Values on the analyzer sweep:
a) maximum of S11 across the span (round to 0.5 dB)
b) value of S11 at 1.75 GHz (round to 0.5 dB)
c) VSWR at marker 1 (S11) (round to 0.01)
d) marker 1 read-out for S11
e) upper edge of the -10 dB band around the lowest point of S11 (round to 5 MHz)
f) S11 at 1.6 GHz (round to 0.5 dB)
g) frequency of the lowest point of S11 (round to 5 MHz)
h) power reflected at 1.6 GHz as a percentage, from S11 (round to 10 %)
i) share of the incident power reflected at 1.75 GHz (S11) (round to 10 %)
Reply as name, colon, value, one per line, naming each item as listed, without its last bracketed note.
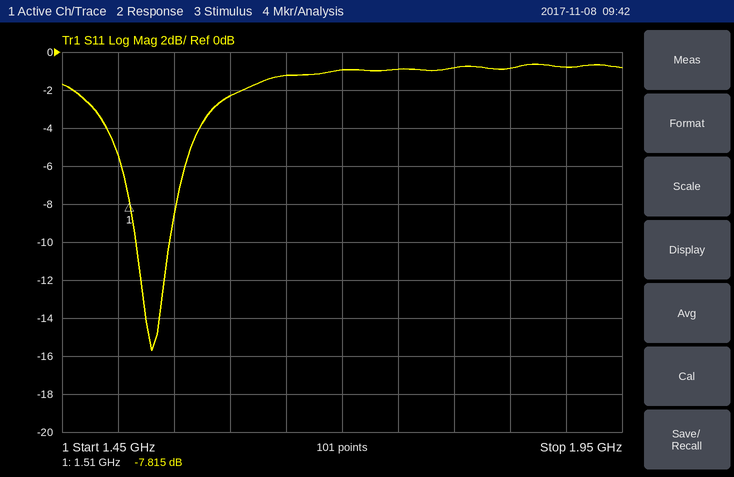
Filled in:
maximum of S11 across the span: -0.5 dB
value of S11 at 1.75 GHz: -1.0 dB
VSWR at marker 1 (S11): 2.37
marker 1 read-out for S11: -7.815 dB
upper edge of the -10 dB band around the lowest point of S11: 1.545 GHz
S11 at 1.6 GHz: -2.5 dB
frequency of the lowest point of S11: 1.530 GHz
power reflected at 1.6 GHz as a percentage, from S11: 60 %
share of the incident power reflected at 1.75 GHz (S11): 80 %
